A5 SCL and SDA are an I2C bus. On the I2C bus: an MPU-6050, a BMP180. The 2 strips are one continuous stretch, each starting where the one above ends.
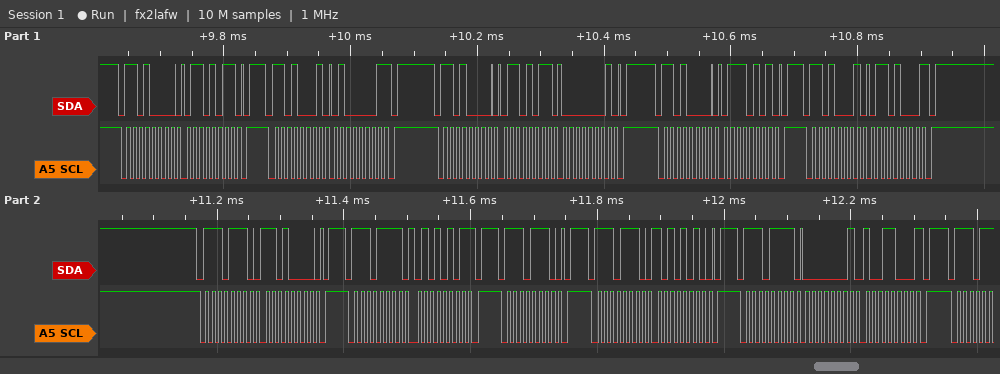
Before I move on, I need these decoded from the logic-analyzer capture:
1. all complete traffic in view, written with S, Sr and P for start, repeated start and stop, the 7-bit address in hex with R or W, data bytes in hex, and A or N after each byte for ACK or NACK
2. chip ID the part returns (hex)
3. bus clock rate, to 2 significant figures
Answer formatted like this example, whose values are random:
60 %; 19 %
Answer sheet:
S 68W A 6B A P S 68R A 41 N P S 68W A 6B A 01 A P S 68W A 75 A P S 68R A 68 N P S 77W A D0 A P S 77R A 55 N P S 77W A P S 77W A AA A P S 77R A 01 A 98 N P; 0x68; 100 kHz
